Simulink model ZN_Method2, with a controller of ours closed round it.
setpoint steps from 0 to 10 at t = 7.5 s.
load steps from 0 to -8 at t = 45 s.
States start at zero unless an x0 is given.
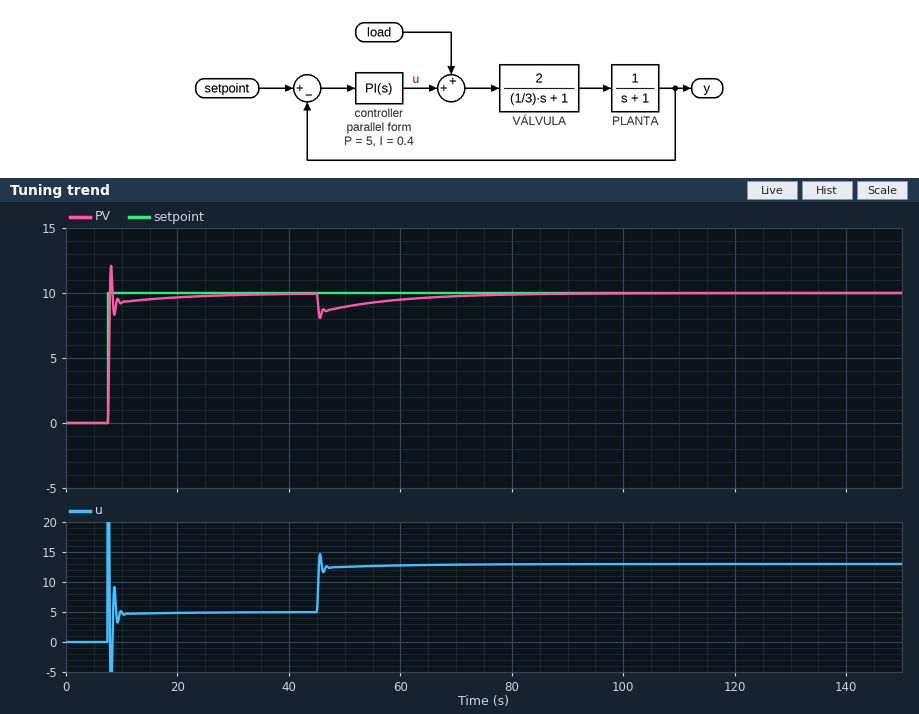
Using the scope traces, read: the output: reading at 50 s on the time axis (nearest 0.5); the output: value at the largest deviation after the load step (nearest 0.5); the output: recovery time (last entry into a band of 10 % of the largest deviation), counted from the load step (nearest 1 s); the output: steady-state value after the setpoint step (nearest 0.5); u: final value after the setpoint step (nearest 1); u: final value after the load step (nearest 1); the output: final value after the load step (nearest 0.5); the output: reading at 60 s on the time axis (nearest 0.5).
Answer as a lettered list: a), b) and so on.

a) 9.0
b) 8.0
c) 29 s
d) 10.0
e) 5
f) 13
g) 10.0
h) 9.5
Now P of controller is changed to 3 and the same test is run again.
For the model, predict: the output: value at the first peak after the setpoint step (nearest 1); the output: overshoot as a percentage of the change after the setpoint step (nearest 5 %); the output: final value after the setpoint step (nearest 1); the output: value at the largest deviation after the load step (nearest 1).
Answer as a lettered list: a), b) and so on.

a) 11
b) 10 %
c) 10
d) 7
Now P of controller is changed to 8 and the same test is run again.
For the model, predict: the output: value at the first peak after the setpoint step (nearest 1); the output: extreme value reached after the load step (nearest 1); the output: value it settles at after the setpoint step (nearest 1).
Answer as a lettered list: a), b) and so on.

a) 13
b) 9
c) 10
